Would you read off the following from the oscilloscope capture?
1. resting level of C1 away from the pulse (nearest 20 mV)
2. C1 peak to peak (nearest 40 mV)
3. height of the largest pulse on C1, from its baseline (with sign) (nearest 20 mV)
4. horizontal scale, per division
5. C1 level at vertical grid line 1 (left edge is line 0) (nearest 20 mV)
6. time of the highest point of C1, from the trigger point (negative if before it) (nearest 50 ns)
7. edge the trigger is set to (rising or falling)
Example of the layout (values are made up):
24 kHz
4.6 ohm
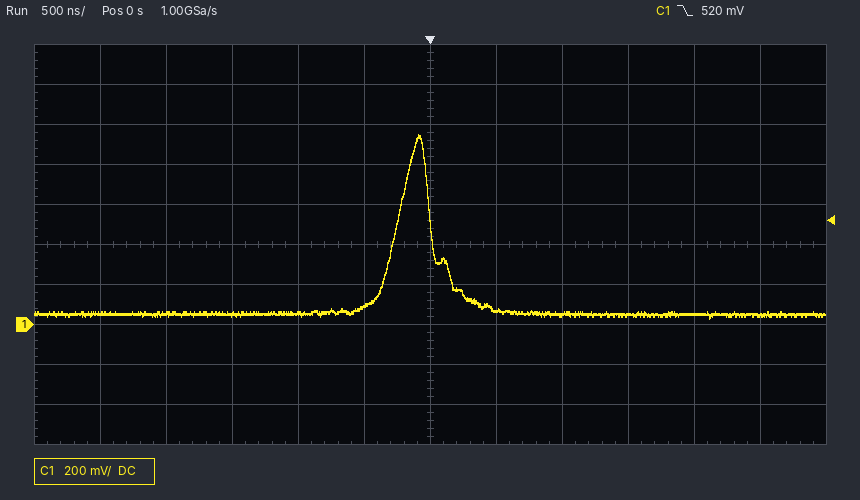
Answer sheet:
60 mV
920 mV
+900 mV
500 ns
60 mV
-100 ns
falling
